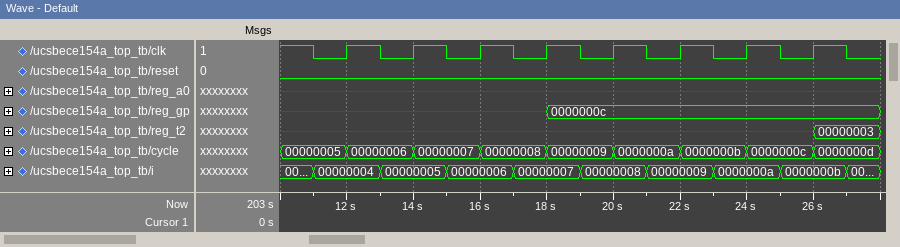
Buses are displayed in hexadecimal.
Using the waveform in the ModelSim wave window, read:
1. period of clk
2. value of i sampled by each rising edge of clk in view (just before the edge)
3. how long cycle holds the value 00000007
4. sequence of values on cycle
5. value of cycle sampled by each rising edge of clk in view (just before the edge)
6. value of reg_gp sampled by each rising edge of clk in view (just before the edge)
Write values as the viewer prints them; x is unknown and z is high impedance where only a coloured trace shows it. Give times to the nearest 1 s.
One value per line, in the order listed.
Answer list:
2 s
00000004, 00000005, 00000006, 00000007, 00000008, 00000009, 0000000a, 0000000b
2 s
00000005, 00000006, 00000007, 00000008, 00000009, 0000000a, 0000000b, 0000000c, 0000000d
00000005, 00000006, 00000007, 00000008, 00000009, 0000000a, 0000000b, 0000000c
x, x, x, x, 0000000c, 0000000c, 0000000c, 0000000c
